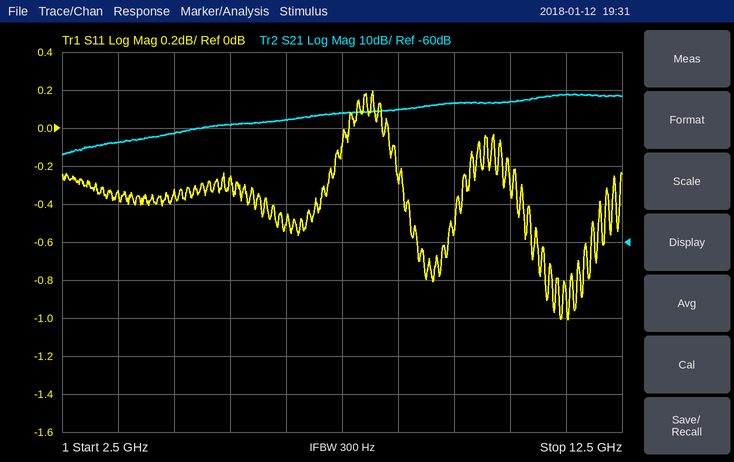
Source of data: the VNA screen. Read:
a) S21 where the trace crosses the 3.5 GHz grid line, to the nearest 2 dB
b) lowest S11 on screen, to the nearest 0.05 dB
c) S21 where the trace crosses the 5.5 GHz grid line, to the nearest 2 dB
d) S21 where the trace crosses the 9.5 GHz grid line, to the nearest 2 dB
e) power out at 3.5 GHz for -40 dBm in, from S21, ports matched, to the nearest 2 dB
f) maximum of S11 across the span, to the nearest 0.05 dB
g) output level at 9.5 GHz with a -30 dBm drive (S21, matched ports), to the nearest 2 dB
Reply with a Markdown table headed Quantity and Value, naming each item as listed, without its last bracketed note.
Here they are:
| Quantity | Value |
|---|---|
| S21 where the trace crosses the 3.5 GHz grid line, to the nearest 2 dB | -34 dB |
| lowest S11 on screen, to the nearest 0.05 dB | -1.00 dB |
| S21 where the trace crosses the 5.5 GHz grid line, to the nearest 2 dB | -30 dB |
| S21 where the trace crosses the 9.5 GHz grid line, to the nearest 2 dB | -24 dB |
| power out at 3.5 GHz for -40 dBm in, from S21, ports matched, to the nearest 2 dB | -74 dBm |
| maximum of S11 across the span, to the nearest 0.05 dB | 0.20 dB |
| output level at 9.5 GHz with a -30 dBm drive (S21, matched ports), to the nearest 2 dB | -54 dBm |
